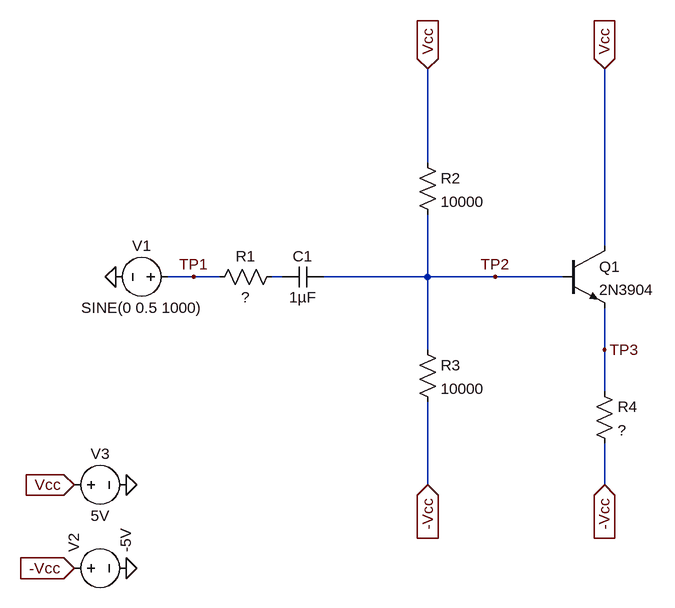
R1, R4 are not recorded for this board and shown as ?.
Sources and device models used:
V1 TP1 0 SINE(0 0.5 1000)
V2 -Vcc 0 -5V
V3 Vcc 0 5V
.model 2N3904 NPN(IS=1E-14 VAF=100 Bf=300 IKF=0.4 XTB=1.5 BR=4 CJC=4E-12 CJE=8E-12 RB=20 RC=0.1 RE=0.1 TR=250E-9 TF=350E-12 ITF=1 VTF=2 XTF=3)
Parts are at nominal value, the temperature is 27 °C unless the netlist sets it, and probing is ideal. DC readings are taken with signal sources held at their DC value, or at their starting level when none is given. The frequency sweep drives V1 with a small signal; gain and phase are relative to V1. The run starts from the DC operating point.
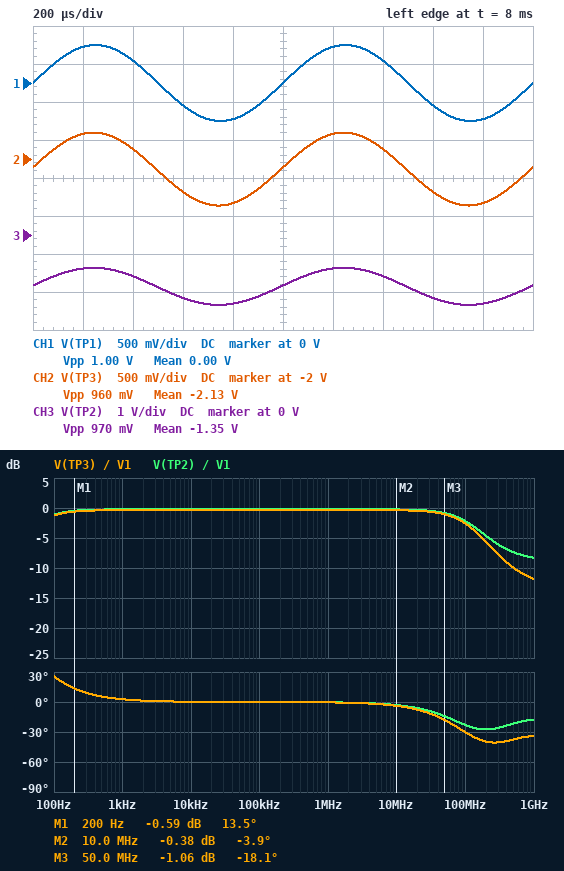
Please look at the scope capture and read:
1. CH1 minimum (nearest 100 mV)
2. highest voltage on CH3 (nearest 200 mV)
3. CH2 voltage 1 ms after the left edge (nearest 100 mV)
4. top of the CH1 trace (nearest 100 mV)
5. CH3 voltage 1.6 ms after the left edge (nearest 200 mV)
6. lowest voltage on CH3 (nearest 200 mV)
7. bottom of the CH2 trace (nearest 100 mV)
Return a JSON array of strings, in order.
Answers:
["-500 mV", "-800 mV", "-2.1 V", "500 mV", "-1.6 V", "-1.8 V", "-2.6 V"]
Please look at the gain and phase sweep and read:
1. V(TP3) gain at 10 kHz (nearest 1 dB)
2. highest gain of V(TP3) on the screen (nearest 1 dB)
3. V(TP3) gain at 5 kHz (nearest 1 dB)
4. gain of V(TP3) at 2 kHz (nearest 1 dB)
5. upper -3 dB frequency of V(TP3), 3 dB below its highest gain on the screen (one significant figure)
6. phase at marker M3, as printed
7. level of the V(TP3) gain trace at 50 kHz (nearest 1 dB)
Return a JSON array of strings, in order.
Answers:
["0 dB", "0 dB", "0 dB", "0 dB", "100 MHz", "-18.1 deg", "0 dB"]
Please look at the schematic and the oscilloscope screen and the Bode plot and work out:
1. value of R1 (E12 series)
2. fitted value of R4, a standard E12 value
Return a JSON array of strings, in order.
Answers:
["82 Ω", "39 Ω"]
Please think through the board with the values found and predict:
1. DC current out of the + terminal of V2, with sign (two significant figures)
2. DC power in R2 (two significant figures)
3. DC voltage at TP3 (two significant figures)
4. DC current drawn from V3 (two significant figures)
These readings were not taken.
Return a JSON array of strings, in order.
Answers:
["-74 mA", "4.0 mW", "-2.1 V", "74 mA"]
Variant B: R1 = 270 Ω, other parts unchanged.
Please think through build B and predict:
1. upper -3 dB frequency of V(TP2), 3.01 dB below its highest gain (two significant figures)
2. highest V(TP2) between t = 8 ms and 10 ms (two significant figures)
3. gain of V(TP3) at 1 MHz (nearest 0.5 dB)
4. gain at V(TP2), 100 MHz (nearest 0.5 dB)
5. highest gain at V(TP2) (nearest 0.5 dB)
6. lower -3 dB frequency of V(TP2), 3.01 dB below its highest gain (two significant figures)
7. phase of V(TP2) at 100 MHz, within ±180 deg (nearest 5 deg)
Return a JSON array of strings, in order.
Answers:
["51 MHz", "-890 mV", "-1.0 dB", "-7.5 dB", "-0.5 dB", "45 Hz", "-45 deg"]
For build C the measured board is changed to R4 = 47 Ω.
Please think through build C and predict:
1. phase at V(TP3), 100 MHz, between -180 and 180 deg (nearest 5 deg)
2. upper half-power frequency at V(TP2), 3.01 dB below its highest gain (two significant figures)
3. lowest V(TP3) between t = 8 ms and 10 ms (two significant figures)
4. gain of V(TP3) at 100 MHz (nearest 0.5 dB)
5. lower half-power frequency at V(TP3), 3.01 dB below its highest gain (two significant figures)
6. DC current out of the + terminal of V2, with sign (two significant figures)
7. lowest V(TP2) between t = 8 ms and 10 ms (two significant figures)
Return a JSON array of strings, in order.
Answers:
["-25 deg", "160 MHz", "-2.4 V", "-2.0 dB", "45 Hz", "-65 mA", "-1.7 V"]
